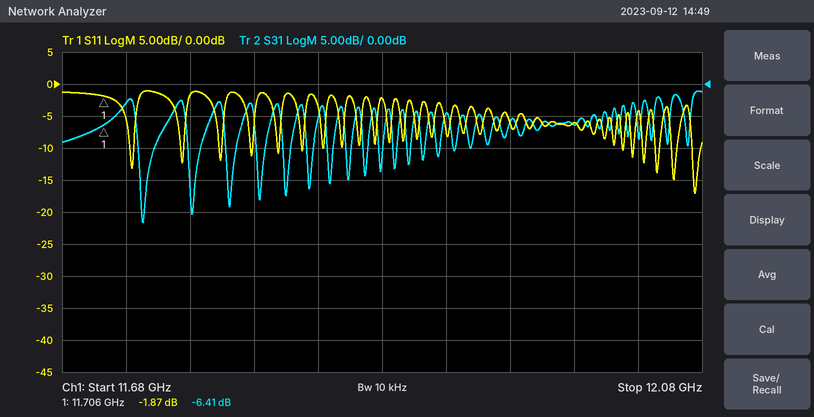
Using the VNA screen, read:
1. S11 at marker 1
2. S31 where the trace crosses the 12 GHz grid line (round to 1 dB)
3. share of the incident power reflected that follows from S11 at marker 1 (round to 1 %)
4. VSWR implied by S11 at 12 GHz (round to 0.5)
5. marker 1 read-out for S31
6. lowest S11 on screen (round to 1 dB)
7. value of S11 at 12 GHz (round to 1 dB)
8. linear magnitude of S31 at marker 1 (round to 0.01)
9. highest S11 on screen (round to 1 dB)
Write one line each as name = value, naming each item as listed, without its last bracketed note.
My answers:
S11 at marker 1 = -1.87 dB
S31 where the trace crosses the 12 GHz grid line = -6 dB
share of the incident power reflected that follows from S11 at marker 1 = 65 %
VSWR implied by S11 at 12 GHz = 3.0
marker 1 read-out for S31 = -6.41 dB
lowest S11 on screen = -17 dB
value of S11 at 12 GHz = -6 dB
linear magnitude of S31 at marker 1 = 0.48
highest S11 on screen = -1 dB
